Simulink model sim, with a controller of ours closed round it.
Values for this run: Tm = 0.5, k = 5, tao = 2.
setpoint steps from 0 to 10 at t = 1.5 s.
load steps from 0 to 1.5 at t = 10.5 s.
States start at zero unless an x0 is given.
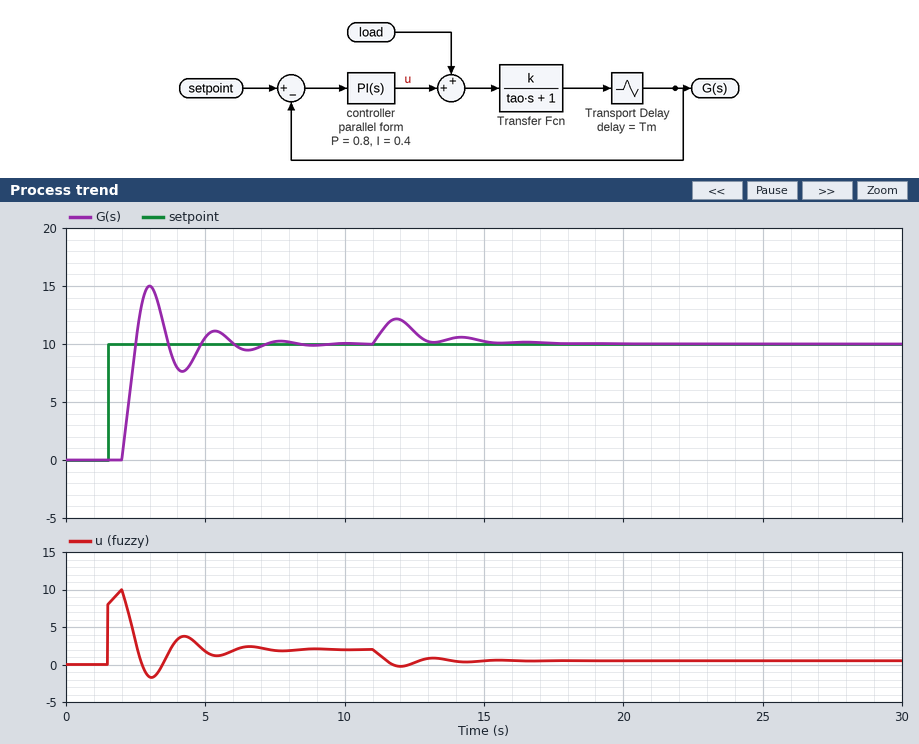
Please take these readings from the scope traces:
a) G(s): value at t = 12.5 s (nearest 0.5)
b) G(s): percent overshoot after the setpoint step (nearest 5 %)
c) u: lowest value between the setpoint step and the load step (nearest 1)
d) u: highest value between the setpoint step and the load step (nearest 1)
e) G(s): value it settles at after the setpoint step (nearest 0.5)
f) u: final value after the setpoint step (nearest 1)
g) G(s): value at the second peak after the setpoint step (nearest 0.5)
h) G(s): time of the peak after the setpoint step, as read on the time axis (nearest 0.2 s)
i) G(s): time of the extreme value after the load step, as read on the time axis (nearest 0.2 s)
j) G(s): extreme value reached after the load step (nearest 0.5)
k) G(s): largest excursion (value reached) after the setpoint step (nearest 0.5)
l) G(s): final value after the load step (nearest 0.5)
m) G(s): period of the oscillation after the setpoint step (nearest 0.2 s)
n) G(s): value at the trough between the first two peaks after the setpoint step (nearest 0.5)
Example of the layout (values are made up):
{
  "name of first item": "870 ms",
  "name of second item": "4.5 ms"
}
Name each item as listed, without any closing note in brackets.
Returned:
{
  "G(s): value at t = 12.5 s": "11.0",
  "G(s): percent overshoot after the setpoint step": "50 %",
  "u: lowest value between the setpoint step and the load step": "-2",
  "u: highest value between the setpoint step and the load step": "10",
  "G(s): value it settles at after the setpoint step": "10.0",
  "u: final value after the setpoint step": "2",
  "G(s): value at the second peak after the setpoint step": "11.0",
  "G(s): time of the peak after the setpoint step, as read on the time axis": "3.0 s",
  "G(s): time of the extreme value after the load step, as read on the time axis": "11.8 s",
  "G(s): extreme value reached after the load step": "12.0",
  "G(s): largest excursion (value reached) after the setpoint step": "15.0",
  "G(s): final value after the load step": "10.0",
  "G(s): period of the oscillation after the setpoint step": "2.4 s",
  "G(s): value at the trough between the first two peaks after the setpoint step": "7.5"
}
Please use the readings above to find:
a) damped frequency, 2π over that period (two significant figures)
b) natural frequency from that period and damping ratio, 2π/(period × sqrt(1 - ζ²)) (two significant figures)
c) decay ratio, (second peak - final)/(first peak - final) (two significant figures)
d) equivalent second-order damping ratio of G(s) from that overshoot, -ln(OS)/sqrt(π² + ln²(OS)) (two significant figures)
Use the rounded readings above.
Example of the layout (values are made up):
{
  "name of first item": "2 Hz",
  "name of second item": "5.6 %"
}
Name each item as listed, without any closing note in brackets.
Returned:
{
  "damped frequency, 2π over that period": "2.6 rad/s",
  "natural frequency from that period and damping ratio, 2π/(period × sqrt(1 - ζ²))": "2.7 rad/s",
  "decay ratio, (second peak - final)/(first peak - final)": "0.20",
  "equivalent second-order damping ratio of G(s) from that overshoot, -ln(OS)/sqrt(π² + ln²(OS))": "0.22"
}
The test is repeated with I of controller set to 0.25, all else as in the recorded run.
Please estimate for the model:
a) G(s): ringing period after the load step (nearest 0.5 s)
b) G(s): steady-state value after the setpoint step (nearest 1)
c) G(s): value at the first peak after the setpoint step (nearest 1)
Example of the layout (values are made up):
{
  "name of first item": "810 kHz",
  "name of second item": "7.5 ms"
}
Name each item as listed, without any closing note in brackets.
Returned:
{
  "G(s): ringing period after the load step": "2.0 s",
  "G(s): steady-state value after the setpoint step": "10",
  "G(s): value at the first peak after the setpoint step": "14"
}
